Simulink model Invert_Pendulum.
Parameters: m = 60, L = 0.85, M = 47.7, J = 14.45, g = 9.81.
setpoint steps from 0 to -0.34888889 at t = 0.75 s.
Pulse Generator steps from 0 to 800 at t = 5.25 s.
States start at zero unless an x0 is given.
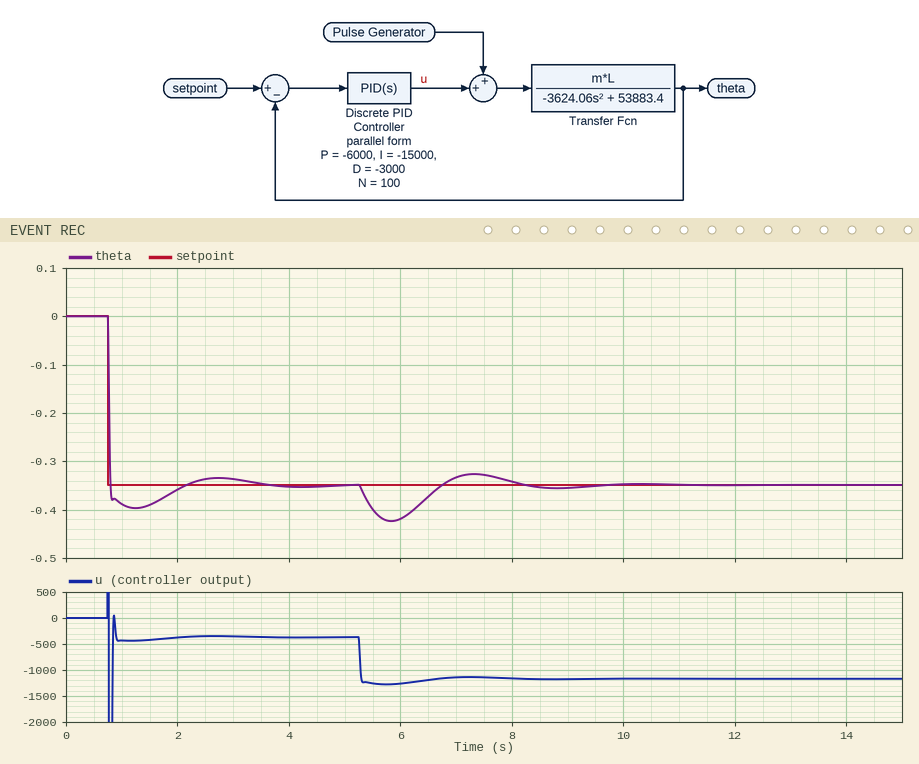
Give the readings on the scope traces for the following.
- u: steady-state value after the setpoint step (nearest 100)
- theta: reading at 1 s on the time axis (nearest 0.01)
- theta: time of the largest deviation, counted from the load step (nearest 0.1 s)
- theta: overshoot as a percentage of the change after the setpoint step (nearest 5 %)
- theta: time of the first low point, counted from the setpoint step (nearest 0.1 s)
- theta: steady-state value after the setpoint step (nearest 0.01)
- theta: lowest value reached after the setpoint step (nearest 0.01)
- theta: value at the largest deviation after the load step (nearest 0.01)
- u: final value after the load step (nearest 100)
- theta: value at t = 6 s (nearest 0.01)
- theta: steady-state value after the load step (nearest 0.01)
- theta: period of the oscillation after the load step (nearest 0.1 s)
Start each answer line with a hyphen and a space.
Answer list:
- -400
- -0.39
- 0.6 s
- 15 %
- 0.5 s
- -0.35
- -0.40
- -0.42
- -1200
- -0.42
- -0.35
- 3.0 s
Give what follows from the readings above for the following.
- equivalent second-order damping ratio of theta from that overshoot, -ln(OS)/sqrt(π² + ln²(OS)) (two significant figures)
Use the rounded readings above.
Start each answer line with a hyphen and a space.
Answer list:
- 0.52
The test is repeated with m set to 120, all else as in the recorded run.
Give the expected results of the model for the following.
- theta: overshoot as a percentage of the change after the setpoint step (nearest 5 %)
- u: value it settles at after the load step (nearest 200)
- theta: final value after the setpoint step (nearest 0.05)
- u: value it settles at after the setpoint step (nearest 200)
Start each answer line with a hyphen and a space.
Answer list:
- 20 %
- -1400
- -0.35
- -600
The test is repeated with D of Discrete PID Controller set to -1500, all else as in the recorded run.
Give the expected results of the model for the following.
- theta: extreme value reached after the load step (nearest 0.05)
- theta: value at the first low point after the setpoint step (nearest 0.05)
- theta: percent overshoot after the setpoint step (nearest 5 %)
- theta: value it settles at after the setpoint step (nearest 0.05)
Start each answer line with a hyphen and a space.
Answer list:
- -0.45
- -0.45
- 25 %
- -0.35
